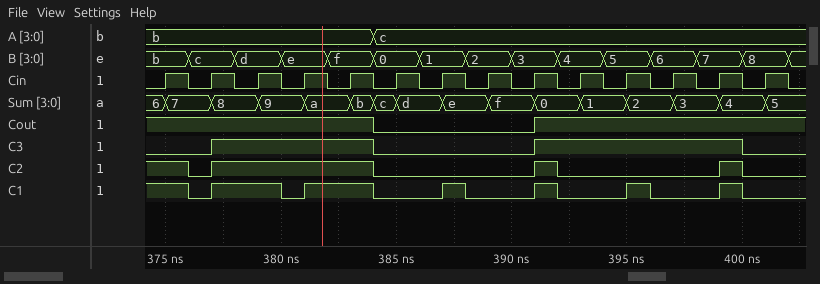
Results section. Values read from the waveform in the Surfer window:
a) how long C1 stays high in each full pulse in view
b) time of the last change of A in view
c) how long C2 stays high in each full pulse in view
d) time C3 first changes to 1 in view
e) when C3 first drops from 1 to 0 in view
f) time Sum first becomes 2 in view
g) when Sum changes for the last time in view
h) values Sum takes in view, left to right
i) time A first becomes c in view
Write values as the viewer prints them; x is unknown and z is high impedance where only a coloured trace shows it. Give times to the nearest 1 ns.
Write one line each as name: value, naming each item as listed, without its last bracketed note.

how long C1 stays high in each full pulse in view: 3 ns, 3 ns, 1 ns, 1 ns, 1 ns, 1 ns
time of the last change of A in view: 384 ns
how long C2 stays high in each full pulse in view: 7 ns, 1 ns, 1 ns
time C3 first changes to 1 in view: 377 ns
when C3 first drops from 1 to 0 in view: 384 ns
time Sum first becomes 2 in view: 395 ns
when Sum changes for the last time in view: 401 ns
values Sum takes in view, left to right: 6, 7, 8, 9, a, b, c, d, e, f, 0, 1, 2, 3, 4, 5
time A first becomes c in view: 384 ns
